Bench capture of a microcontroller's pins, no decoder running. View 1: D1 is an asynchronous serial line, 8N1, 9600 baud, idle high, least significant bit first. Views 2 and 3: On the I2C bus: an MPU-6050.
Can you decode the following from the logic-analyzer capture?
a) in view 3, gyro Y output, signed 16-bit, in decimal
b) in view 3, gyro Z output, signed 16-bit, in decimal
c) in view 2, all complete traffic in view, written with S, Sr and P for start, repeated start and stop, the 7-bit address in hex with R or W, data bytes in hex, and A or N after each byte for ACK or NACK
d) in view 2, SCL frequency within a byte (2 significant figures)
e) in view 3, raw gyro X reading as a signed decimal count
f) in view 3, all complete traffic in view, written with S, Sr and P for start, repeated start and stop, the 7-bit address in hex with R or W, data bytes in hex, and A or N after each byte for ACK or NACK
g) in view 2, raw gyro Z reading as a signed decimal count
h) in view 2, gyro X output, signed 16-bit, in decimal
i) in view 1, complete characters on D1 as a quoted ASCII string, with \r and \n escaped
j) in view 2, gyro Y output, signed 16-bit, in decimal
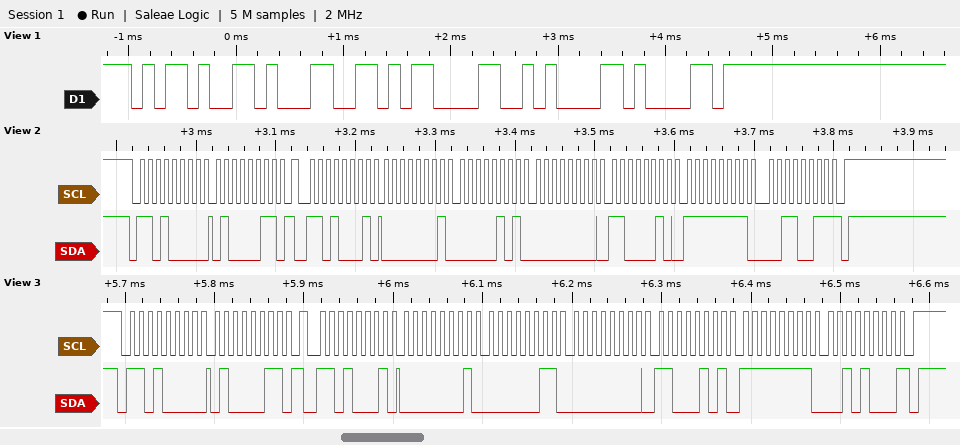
197
-216
S 68W A 43 A Sr 68R A 01 A 05 A 00 A C2 A FF A 33 N P
100 kHz
259
S 68W A 43 A Sr 68R A 01 A 03 A 00 A C5 A FF A 28 N P
-205
261
"-1\r\na"
194
